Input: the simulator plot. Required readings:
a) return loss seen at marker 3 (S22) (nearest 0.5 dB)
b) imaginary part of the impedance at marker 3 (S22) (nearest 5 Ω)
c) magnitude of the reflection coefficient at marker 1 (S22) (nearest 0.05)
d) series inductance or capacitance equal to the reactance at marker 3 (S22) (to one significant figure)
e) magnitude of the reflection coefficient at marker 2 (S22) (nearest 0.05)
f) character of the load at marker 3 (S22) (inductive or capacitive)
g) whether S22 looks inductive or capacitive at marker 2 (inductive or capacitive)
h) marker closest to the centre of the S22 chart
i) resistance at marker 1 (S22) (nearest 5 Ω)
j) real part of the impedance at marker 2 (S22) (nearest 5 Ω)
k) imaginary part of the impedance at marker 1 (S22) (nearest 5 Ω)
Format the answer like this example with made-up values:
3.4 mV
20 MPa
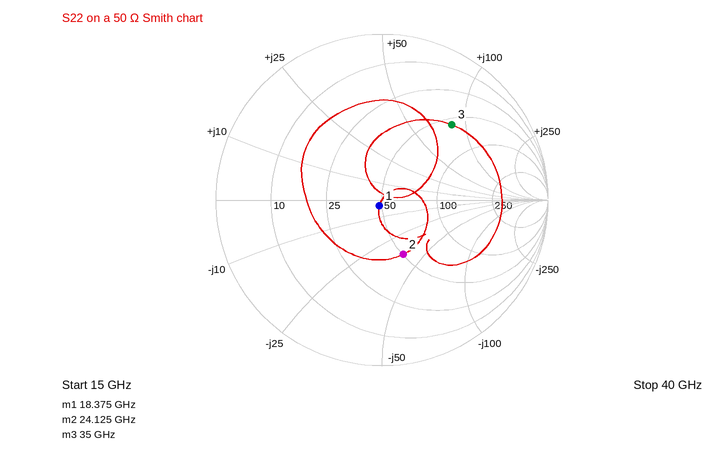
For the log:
4.0 dB
+85 Ω
0.05
400 pH
0.35
inductive
capacitive
marker 1
50 Ω
50 Ω
-5 Ω
